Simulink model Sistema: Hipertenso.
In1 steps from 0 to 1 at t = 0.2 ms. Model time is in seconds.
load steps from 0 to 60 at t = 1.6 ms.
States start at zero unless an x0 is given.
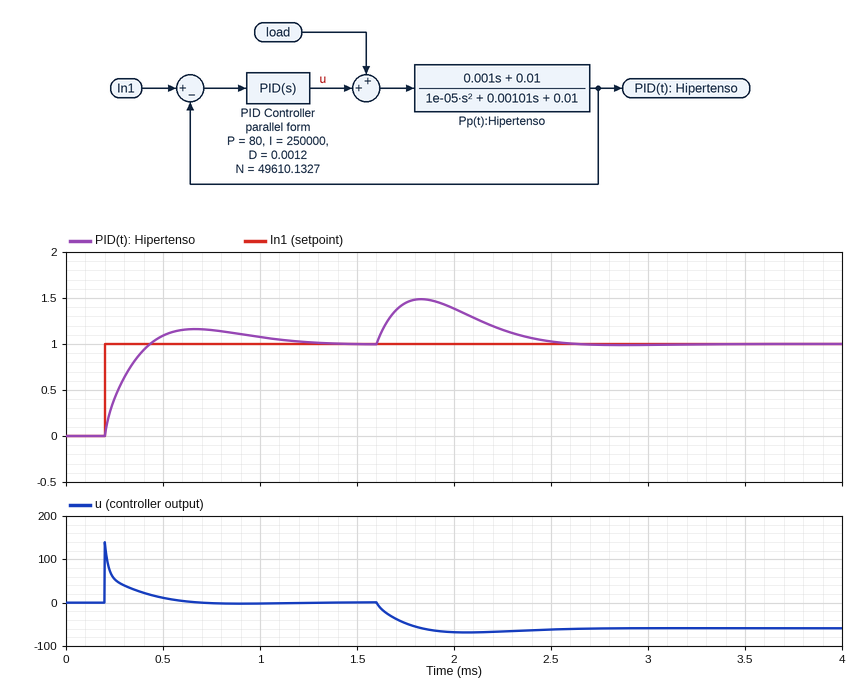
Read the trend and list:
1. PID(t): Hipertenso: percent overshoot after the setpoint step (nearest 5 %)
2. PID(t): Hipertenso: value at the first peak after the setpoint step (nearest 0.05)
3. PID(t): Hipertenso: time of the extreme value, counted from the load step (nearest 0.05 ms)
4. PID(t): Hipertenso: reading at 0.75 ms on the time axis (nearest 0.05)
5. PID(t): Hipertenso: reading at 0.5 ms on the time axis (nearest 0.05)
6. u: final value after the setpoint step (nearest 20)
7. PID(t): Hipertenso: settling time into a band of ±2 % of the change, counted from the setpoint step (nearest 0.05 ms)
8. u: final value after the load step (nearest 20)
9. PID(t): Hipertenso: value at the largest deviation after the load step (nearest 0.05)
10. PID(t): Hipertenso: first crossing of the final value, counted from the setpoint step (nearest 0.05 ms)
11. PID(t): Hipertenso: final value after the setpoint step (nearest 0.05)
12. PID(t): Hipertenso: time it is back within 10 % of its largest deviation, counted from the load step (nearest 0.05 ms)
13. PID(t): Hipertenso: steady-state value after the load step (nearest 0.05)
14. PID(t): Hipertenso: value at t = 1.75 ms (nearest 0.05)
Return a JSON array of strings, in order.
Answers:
["15 %", "1.15", "0.25 ms", "1.15", "1.10", "0", "1.05 ms", "-60", "1.50", "0.25 ms", "1.00", "0.85 ms", "1.00", "1.45"]
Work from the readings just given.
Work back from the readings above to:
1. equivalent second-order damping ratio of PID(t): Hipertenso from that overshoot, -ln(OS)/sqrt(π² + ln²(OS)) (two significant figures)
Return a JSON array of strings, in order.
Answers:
["0.52"]
